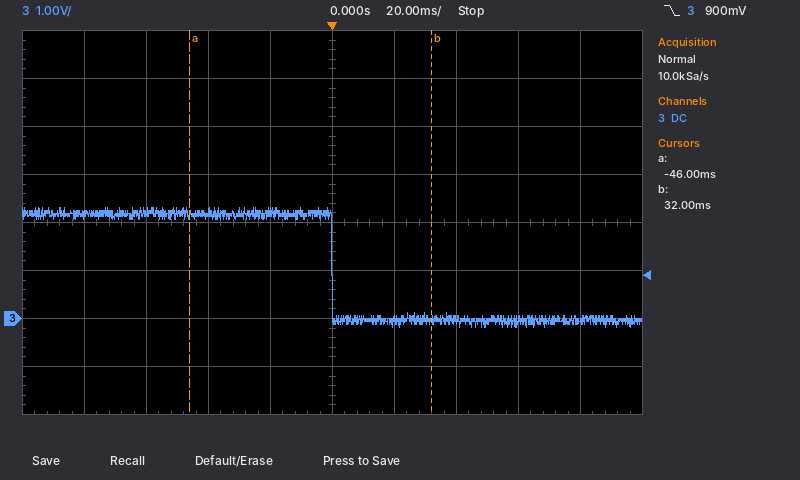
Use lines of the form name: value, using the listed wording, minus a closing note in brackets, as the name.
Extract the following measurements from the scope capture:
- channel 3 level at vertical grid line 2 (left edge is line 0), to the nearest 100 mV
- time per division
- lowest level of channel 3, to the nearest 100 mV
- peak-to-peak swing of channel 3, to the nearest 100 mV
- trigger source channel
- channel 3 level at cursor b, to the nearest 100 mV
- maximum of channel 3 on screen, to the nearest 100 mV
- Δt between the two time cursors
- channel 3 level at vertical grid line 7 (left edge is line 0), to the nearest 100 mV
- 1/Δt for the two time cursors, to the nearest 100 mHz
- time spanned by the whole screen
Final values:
channel 3 level at vertical grid line 2 (left edge is line 0), to the nearest 100 mV: 2.2 V
time per division: 20 ms
lowest level of channel 3, to the nearest 100 mV: -200 mV
peak-to-peak swing of channel 3, to the nearest 100 mV: 2.5 V
trigger source channel: channel 3
channel 3 level at cursor b, to the nearest 100 mV: 0.0 V
maximum of channel 3 on screen, to the nearest 100 mV: 2.3 V
Δt between the two time cursors: 78 ms
channel 3 level at vertical grid line 7 (left edge is line 0), to the nearest 100 mV: 0.0 V
1/Δt for the two time cursors, to the nearest 100 mHz: 12.8 Hz
time spanned by the whole screen: 200 ms
